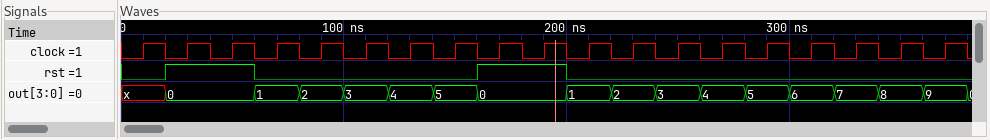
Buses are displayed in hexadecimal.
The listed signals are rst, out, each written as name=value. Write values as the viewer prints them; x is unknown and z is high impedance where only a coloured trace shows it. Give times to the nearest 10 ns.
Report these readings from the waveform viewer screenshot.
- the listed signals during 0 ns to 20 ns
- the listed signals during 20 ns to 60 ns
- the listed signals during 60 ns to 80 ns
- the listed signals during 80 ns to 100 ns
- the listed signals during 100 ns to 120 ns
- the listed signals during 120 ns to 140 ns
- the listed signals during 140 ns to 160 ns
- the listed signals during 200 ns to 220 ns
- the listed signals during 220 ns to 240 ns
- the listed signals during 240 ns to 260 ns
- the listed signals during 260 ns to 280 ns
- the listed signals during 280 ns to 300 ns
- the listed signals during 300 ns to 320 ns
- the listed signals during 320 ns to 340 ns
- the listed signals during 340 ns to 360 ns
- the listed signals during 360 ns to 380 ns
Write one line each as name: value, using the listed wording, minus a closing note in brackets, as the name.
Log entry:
the listed signals during 0 ns to 20 ns: rst=0, out=x
the listed signals during 20 ns to 60 ns: rst=1, out=0
the listed signals during 60 ns to 80 ns: rst=0, out=1
the listed signals during 80 ns to 100 ns: rst=0, out=2
the listed signals during 100 ns to 120 ns: rst=0, out=3
the listed signals during 120 ns to 140 ns: rst=0, out=4
the listed signals during 140 ns to 160 ns: rst=0, out=5
the listed signals during 200 ns to 220 ns: rst=0, out=1
the listed signals during 220 ns to 240 ns: rst=0, out=2
the listed signals during 240 ns to 260 ns: rst=0, out=3
the listed signals during 260 ns to 280 ns: rst=0, out=4
the listed signals during 280 ns to 300 ns: rst=0, out=5
the listed signals during 300 ns to 320 ns: rst=0, out=6
the listed signals during 320 ns to 340 ns: rst=0, out=7
the listed signals during 340 ns to 360 ns: rst=0, out=8
the listed signals during 360 ns to 380 ns: rst=0, out=9
